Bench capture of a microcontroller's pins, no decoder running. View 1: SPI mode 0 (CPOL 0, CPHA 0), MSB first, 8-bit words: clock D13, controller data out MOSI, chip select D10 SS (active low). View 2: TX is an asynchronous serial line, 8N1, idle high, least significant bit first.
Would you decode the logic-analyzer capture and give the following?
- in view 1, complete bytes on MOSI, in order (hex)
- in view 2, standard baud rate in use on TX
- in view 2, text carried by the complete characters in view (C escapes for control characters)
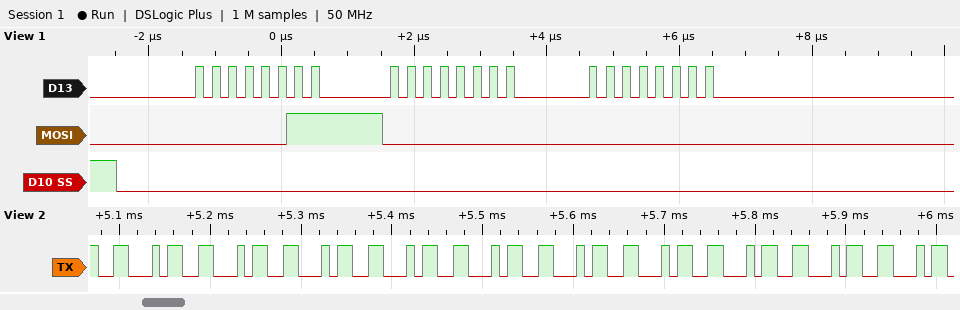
03 00 00
115200 baud
"FFFFFFFFFF"
